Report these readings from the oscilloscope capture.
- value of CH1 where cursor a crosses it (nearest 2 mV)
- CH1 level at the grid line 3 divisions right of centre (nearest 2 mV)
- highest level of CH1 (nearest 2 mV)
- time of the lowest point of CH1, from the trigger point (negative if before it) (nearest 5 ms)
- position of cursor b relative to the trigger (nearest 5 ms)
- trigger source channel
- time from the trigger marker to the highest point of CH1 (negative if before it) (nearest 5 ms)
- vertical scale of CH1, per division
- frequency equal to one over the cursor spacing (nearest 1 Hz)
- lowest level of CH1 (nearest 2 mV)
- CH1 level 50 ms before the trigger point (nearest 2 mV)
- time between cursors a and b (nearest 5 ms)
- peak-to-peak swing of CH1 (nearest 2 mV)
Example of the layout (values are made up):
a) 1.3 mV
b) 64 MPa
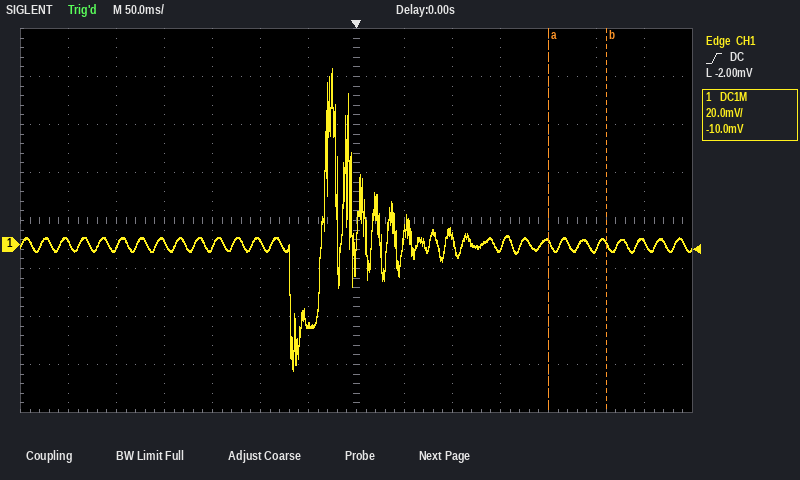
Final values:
a) 0 mV
b) -2 mV
c) 74 mV
d) -65 ms
e) +260 ms
f) CH1
g) -25 ms
h) 20 mV
i) 17 Hz
j) -52 mV
k) -34 mV
l) 60 ms
m) 126 mV
